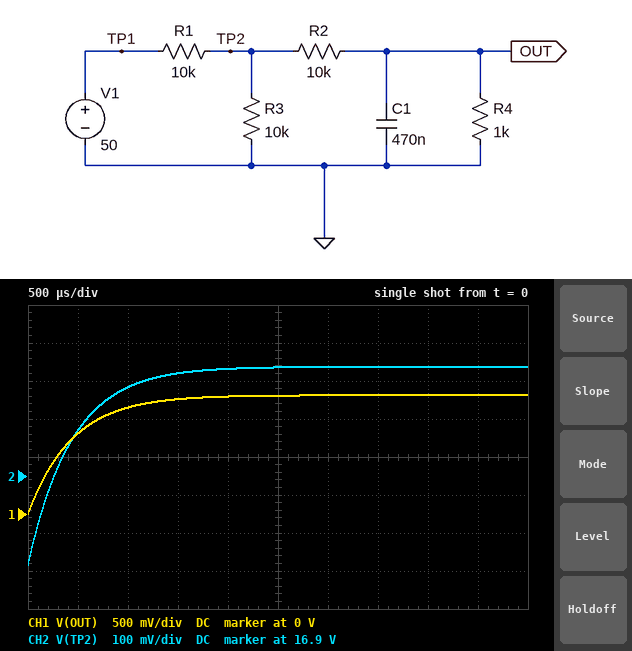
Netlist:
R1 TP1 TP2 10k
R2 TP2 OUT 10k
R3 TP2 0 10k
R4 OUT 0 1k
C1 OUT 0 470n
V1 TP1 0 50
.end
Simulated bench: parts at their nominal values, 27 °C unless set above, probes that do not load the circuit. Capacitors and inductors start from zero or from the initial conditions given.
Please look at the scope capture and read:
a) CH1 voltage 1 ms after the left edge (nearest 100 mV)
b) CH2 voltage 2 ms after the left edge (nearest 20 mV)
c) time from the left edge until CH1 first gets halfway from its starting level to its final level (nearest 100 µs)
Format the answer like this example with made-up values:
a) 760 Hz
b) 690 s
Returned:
a) 1.4 V
b) 17.18 V
c) 300 µs
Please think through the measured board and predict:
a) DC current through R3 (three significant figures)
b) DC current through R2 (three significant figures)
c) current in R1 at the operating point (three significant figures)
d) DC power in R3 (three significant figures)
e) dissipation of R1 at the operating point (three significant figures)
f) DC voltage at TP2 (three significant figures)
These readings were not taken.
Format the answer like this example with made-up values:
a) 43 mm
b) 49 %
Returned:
a) 1.72 mA
b) 1.56 mA
c) 3.28 mA
d) 29.5 mW
e) 108 mW
f) 17.2 V
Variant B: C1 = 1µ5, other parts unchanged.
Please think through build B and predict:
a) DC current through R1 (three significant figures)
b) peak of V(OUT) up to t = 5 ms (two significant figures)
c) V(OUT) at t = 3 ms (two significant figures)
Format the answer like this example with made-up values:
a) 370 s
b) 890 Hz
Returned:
a) 3.28 mA
b) 1.5 V
c) 1.4 V
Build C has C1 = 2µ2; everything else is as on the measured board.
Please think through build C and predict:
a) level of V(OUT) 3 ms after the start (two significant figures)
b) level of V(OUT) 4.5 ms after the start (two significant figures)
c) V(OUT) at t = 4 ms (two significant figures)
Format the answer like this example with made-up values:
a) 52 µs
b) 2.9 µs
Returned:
a) 1.2 V
b) 1.4 V
c) 1.3 V
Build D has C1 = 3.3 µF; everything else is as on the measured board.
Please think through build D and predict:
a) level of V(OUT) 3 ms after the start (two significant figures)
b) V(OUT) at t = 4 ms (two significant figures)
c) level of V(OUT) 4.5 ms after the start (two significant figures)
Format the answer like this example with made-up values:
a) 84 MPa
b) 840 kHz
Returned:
a) 970 mV
b) 1.1 V
c) 1.2 V
